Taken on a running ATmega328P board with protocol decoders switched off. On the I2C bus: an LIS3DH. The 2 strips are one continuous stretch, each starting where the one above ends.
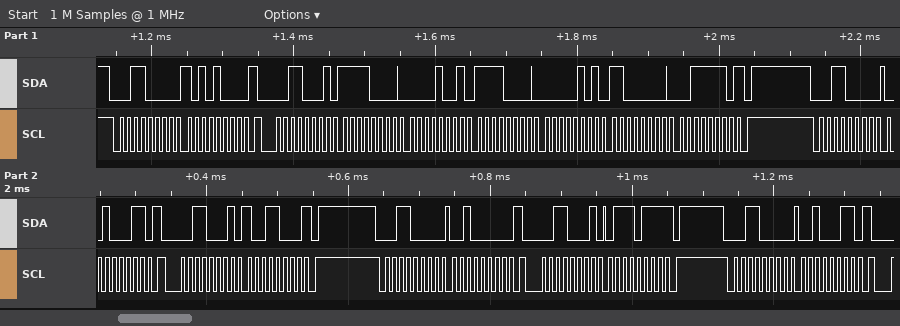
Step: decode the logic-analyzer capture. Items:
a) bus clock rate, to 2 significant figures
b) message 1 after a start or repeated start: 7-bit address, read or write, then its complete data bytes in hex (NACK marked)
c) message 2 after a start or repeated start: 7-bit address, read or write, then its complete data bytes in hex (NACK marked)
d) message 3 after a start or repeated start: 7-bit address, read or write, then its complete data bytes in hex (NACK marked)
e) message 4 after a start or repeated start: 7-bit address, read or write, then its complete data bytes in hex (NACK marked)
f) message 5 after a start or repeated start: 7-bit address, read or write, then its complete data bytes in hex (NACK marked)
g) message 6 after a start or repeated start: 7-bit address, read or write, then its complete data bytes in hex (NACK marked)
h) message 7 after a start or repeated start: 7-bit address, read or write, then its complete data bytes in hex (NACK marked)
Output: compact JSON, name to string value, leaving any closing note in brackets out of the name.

{"bus clock rate, to 2 significant figures": "100 kHz", "message 1 after a start or repeated start: 7-bit address, read or write, then its complete data bytes in hex": "0x18 write: A8", "message 2 after a start or repeated start: 7-bit address, read or write, then its complete data bytes in hex": "0x18 read: F0 09 F0 05 C0 3E NACK", "message 3 after a start or repeated start: 7-bit address, read or write, then its complete data bytes in hex": "0x18 write: 23", "message 4 after a start or repeated start: 7-bit address, read or write, then its complete data bytes in hex": "0x18 read: 98 NACK", "message 5 after a start or repeated start: 7-bit address, read or write, then its complete data bytes in hex": "0x18 write: 20", "message 6 after a start or repeated start: 7-bit address, read or write, then its complete data bytes in hex": "0x18 read: 77 NACK", "message 7 after a start or repeated start: 7-bit address, read or write, then its complete data bytes in hex": "0x18 write: 23"}
